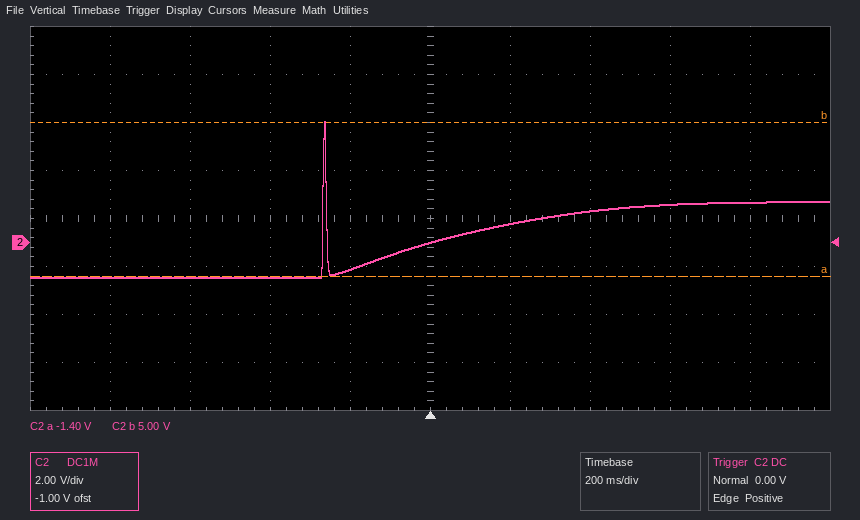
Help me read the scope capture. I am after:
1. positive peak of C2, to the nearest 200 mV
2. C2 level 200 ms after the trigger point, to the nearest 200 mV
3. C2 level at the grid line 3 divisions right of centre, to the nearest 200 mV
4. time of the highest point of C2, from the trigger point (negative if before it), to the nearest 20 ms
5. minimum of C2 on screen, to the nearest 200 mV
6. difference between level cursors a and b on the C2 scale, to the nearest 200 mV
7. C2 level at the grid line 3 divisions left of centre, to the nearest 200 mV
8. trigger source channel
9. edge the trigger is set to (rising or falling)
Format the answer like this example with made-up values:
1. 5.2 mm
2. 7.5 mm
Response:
1. 5.0 V
2. 800 mV
3. 1.6 V
4. -260 ms
5. -1.4 V
6. 6.4 V
7. -1.4 V
8. C2
9. rising
